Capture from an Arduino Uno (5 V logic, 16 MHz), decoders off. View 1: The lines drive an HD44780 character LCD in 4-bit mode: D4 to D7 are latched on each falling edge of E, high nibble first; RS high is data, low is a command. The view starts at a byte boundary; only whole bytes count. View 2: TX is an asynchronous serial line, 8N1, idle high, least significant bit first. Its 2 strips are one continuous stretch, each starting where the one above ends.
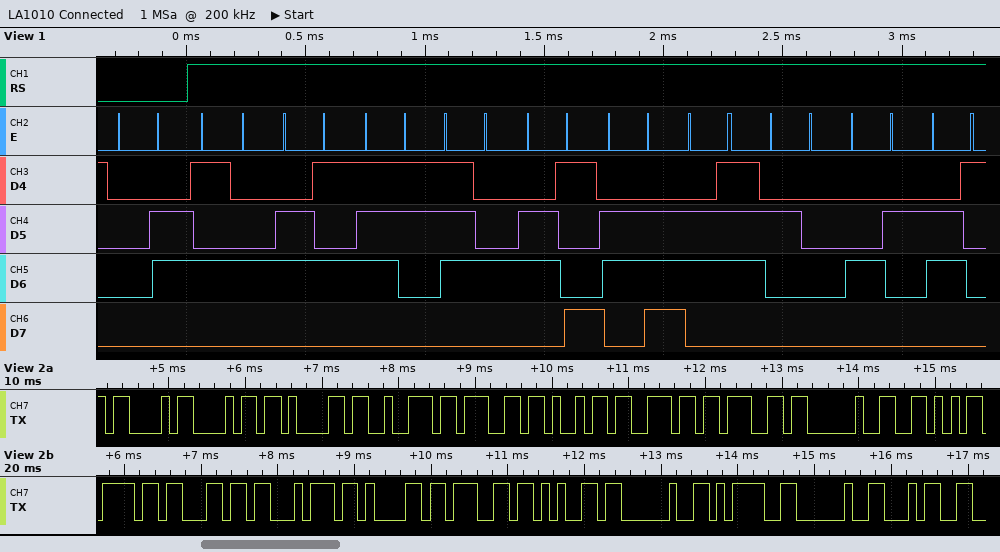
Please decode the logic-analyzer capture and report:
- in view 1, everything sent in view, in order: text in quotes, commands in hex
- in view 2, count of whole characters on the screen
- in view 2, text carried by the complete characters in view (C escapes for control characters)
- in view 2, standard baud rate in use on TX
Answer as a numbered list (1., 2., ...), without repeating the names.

1. 0x06 "Testing Ba"
2. 20
3. "Charging Voltage = 4"
4. 9600 baud
